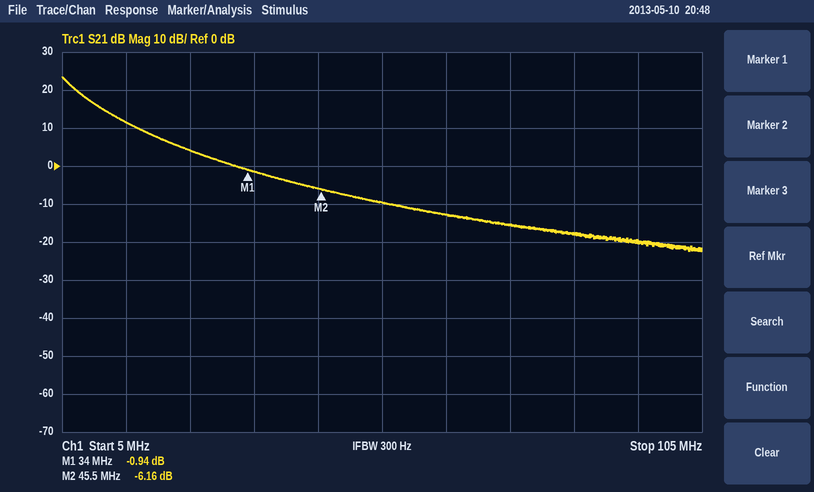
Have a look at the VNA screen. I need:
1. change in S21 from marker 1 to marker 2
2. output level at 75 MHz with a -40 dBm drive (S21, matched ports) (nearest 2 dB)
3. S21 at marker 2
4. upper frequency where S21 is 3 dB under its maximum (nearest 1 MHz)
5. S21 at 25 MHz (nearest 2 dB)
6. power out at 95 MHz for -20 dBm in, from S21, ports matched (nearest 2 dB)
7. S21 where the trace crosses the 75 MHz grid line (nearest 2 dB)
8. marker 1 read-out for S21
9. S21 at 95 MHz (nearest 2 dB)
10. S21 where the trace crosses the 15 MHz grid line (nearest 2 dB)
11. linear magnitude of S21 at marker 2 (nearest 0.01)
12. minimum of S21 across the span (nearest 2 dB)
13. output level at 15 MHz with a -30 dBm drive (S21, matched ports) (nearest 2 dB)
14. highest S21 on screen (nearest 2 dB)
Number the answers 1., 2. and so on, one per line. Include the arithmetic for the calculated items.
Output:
1. -6.16 − (-0.94) = -5.22 dB
2. -40 dBm + (-16 dB) = -56 dBm
3. -6.16 dB
4. 7 MHz
5. 4 dB
6. -20 dBm + (-20 dB) = -40 dBm
7. -16 dB
8. -0.94 dB
9. -20 dB
10. 12 dB
11. 10^(-6.16/20) ≈ 0.49
12. -22 dB
13. -30 dBm + (12 dB) = -18 dBm
14. 24 dB
